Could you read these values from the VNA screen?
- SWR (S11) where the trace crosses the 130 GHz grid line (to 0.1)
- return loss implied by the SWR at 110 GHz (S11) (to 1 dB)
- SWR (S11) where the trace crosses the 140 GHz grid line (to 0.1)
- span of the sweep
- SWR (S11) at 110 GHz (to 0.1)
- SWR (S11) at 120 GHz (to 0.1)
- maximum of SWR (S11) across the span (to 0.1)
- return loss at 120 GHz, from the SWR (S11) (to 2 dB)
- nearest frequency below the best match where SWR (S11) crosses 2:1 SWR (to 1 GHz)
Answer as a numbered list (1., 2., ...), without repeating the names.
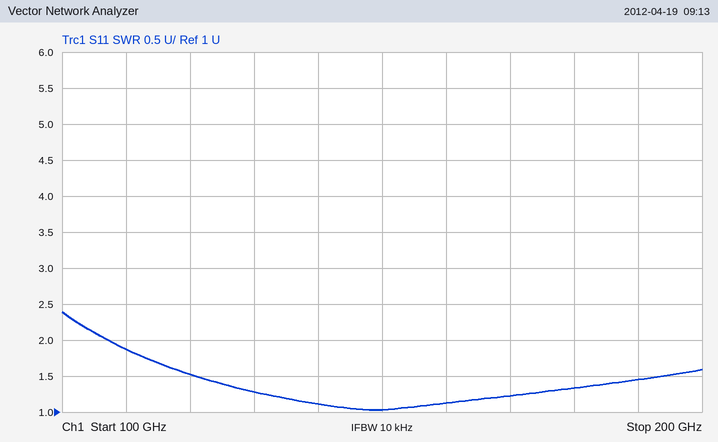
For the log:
1. 1.3
2. 10 dB
3. 1.1
4. 100 GHz
5. 1.9
6. 1.5
7. 2.4
8. 14 dB
9. 107 GHz
